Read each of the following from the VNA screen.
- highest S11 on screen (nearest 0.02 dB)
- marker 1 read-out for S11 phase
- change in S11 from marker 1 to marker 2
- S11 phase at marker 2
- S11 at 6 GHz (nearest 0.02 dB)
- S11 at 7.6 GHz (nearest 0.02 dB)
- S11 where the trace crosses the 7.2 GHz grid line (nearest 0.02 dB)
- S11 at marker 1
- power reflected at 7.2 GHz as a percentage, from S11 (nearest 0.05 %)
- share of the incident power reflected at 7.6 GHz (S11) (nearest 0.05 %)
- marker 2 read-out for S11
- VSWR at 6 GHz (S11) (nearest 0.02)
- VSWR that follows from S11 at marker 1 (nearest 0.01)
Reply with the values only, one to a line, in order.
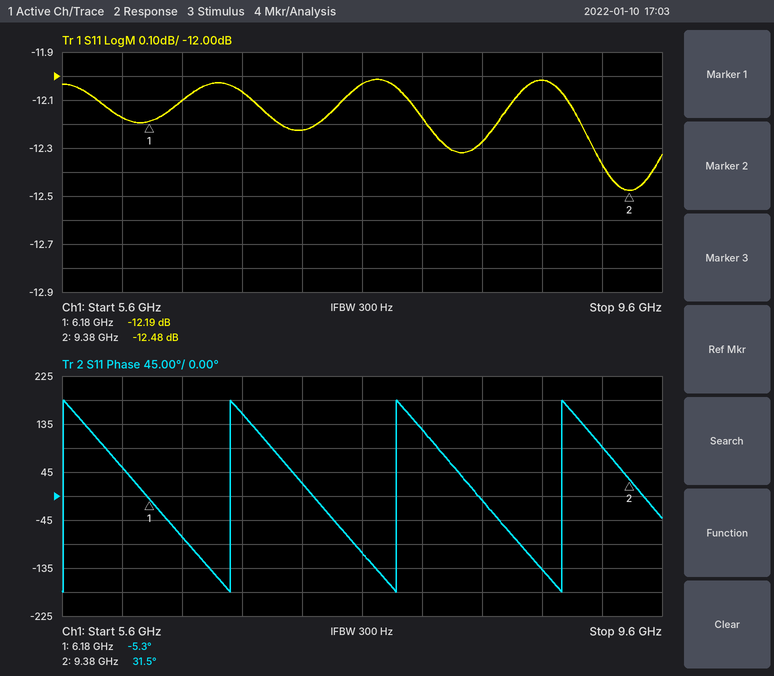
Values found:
-12.02 dB
-5.3°
-0.29 dB
31.5°
-12.18 dB
-12.04 dB
-12.22 dB
-12.19 dB
6.00 %
6.25 %
-12.48 dB
1.66
1.65
